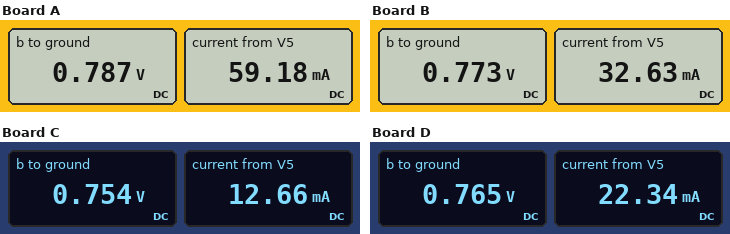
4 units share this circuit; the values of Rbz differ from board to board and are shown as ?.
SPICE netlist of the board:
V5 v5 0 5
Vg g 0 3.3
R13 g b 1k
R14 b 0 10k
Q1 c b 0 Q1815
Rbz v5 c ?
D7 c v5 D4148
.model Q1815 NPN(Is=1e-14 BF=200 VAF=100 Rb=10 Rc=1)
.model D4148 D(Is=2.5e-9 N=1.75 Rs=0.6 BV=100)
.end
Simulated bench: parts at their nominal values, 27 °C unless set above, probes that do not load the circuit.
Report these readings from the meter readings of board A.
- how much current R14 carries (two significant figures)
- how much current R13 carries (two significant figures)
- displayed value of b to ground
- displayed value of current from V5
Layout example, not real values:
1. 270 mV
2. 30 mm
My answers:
1. 79 µA
2. 2.5 mA
3. 0.787 V
4. 59.18 mA
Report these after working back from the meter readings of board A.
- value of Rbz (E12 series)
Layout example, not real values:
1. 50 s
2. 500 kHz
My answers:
1. 82 Ω
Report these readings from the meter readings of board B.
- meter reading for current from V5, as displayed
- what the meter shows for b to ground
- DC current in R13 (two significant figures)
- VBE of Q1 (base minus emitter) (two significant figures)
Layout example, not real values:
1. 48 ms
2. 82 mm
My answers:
1. 32.63 mA
2. 0.773 V
3. 2.5 mA
4. 770 mV
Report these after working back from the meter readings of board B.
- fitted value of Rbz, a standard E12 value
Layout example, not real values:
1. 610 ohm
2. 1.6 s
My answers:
1. 150 Ω
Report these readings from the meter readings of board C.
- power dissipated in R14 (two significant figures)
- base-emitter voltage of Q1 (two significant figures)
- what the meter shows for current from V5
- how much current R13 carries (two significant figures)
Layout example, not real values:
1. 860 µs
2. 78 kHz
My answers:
1. 57 µW
2. 750 mV
3. 12.66 mA
4. 2.5 mA
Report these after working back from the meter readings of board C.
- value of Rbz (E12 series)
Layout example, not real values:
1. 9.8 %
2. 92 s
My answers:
1. 390 Ω
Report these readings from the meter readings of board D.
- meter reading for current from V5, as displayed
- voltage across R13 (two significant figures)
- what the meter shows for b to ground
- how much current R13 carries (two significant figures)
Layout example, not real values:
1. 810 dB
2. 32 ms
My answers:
1. 22.34 mA
2. 2.5 V
3. 0.765 V
4. 2.5 mA
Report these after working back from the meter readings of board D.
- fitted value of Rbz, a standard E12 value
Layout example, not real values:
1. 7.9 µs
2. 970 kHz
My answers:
1. 220 Ω
